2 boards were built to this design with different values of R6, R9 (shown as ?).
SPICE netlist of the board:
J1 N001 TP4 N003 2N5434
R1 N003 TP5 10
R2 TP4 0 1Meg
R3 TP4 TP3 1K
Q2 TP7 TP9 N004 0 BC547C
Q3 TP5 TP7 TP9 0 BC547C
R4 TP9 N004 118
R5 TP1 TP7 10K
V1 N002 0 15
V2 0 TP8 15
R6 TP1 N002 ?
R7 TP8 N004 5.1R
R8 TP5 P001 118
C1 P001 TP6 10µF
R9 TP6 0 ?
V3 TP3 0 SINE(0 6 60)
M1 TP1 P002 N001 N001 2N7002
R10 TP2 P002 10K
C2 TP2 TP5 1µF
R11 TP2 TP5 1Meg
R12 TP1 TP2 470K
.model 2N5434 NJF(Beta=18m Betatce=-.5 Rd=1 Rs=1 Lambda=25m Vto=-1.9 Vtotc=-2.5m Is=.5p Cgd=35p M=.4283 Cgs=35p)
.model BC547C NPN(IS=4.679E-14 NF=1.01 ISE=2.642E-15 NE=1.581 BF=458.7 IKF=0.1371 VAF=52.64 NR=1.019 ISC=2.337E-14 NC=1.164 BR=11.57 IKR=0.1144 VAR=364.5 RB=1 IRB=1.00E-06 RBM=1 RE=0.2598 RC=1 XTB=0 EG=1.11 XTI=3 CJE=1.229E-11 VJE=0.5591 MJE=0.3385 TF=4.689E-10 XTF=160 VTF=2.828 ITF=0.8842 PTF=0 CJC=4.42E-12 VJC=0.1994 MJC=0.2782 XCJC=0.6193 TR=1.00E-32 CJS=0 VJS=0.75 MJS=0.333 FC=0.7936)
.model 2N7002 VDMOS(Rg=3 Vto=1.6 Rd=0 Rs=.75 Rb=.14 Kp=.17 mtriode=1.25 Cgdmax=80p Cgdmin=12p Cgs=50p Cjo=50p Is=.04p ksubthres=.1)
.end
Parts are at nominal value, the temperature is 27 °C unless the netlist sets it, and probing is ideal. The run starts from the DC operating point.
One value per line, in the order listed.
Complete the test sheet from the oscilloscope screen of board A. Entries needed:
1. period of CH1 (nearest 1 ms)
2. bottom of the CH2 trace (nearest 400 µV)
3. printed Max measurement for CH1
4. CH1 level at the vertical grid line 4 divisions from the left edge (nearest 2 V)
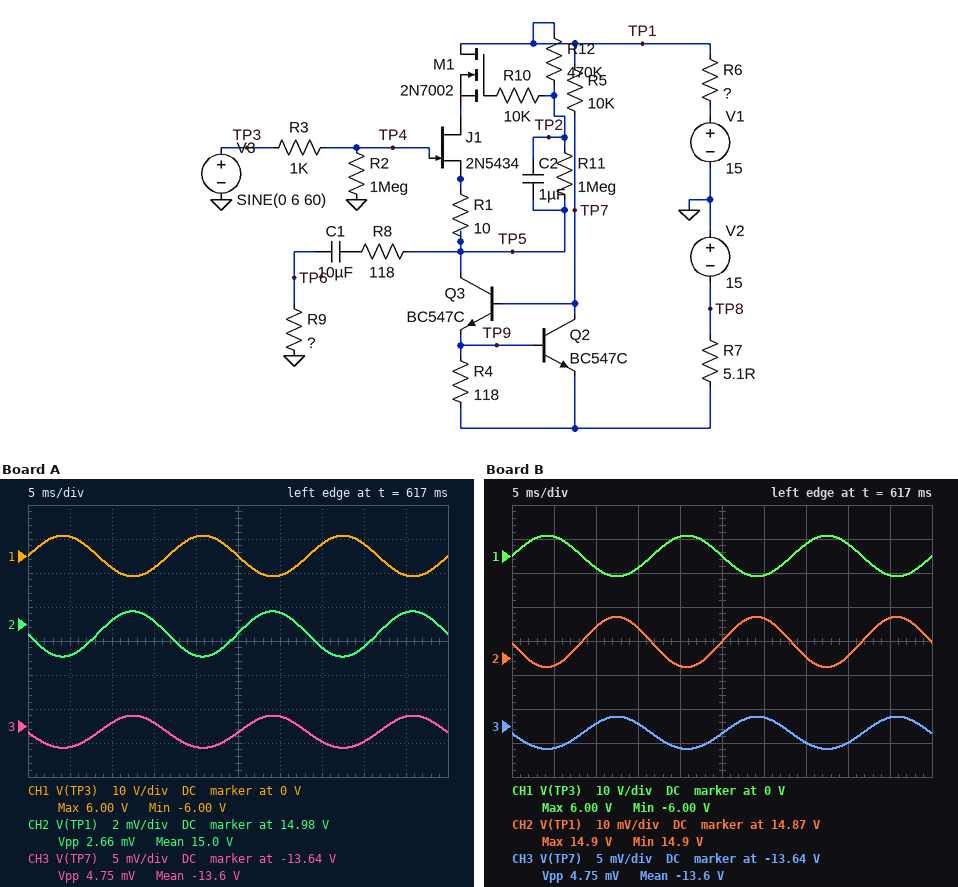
17 ms
14.9760 V
6.00 V
6 V
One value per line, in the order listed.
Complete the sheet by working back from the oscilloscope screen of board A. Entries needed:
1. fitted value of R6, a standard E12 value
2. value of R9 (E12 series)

2.7 Ω
12 kΩ
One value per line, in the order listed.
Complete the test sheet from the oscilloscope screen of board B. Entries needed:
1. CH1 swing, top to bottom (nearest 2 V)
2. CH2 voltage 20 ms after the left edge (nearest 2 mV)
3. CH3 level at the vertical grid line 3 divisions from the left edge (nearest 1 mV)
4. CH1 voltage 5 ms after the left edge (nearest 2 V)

12 V
14.868 V
-13.645 V
6 V
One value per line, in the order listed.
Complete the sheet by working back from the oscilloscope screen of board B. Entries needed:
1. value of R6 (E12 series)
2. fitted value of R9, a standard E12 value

15 Ω
12 kΩ
